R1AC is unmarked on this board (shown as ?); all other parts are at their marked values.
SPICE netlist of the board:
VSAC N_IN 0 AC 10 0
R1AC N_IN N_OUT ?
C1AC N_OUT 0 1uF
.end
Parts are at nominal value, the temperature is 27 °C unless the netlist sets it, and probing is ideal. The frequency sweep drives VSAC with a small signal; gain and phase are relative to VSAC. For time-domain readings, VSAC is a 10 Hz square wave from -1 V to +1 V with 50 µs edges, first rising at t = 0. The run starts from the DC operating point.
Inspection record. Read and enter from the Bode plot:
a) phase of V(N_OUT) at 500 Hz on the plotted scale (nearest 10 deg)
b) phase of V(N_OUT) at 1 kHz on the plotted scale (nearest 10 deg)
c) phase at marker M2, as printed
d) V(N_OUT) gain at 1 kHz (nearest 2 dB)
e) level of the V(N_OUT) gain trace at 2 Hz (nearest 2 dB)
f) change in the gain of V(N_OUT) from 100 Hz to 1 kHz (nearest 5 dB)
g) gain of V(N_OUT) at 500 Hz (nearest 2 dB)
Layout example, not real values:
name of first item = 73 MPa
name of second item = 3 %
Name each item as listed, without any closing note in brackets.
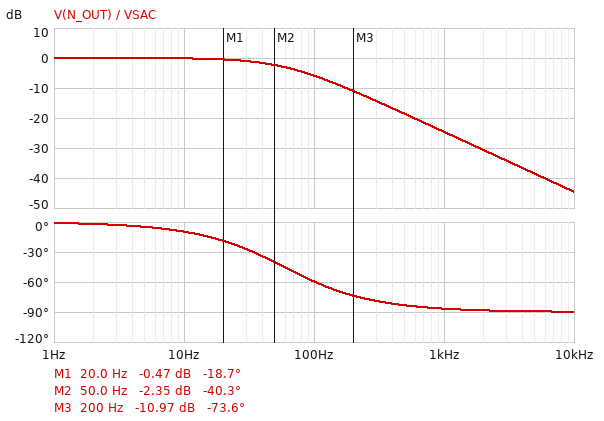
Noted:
phase of V(N_OUT) at 500 Hz on the plotted scale = -80 deg
phase of V(N_OUT) at 1 kHz on the plotted scale = -90 deg
phase at marker M2, as printed = -40.3 deg
V(N_OUT) gain at 1 kHz = -24 dB
level of the V(N_OUT) gain trace at 2 Hz = 0 dB
change in the gain of V(N_OUT) from 100 Hz to 1 kHz = -20 dB
gain of V(N_OUT) at 500 Hz = -18 dB
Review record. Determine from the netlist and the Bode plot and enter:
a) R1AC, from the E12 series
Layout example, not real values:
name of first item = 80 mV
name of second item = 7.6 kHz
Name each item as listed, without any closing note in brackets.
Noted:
R1AC, from the E12 series = 2.7 kΩ
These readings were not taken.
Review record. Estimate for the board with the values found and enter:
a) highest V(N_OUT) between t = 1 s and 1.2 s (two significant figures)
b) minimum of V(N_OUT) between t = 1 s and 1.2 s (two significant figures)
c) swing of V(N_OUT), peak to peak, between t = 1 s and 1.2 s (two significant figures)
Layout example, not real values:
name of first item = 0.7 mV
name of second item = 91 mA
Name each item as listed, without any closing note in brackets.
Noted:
highest V(N_OUT) between t = 1 s and 1.2 s = 1.0 V
minimum of V(N_OUT) between t = 1 s and 1.2 s = -1.0 V
swing of V(N_OUT), peak to peak, between t = 1 s and 1.2 s = 2.0 V
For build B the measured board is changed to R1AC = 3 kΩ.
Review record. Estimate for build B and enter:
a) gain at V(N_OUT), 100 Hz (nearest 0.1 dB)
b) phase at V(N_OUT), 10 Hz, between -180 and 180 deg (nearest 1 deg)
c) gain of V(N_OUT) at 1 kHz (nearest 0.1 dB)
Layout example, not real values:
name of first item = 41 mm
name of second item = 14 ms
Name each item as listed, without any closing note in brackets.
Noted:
gain at V(N_OUT), 100 Hz = -6.6 dB
phase at V(N_OUT), 10 Hz, between -180 and 180 deg = -11 deg
gain of V(N_OUT) at 1 kHz = -25.5 dB
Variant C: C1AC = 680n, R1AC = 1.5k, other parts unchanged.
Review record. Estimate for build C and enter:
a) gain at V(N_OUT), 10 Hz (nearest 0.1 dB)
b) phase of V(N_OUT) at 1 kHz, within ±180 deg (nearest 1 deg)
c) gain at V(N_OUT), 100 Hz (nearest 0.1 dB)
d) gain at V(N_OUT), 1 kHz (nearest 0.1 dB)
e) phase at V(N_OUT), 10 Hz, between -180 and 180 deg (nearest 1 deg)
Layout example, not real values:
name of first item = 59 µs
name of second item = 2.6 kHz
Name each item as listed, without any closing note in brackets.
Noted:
gain at V(N_OUT), 10 Hz = 0 dB
phase of V(N_OUT) at 1 kHz, within ±180 deg = -81 deg
gain at V(N_OUT), 100 Hz = -1.5 dB
gain at V(N_OUT), 1 kHz = -16.2 dB
phase at V(N_OUT), 10 Hz, between -180 and 180 deg = -4 deg
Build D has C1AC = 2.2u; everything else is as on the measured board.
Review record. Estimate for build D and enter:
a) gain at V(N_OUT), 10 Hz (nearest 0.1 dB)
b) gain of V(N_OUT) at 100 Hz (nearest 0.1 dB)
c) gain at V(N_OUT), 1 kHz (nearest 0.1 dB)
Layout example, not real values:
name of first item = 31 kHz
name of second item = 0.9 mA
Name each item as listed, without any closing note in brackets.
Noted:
gain at V(N_OUT), 10 Hz = -0.6 dB
gain of V(N_OUT) at 100 Hz = -11.7 dB
gain at V(N_OUT), 1 kHz = -31.4 dB
